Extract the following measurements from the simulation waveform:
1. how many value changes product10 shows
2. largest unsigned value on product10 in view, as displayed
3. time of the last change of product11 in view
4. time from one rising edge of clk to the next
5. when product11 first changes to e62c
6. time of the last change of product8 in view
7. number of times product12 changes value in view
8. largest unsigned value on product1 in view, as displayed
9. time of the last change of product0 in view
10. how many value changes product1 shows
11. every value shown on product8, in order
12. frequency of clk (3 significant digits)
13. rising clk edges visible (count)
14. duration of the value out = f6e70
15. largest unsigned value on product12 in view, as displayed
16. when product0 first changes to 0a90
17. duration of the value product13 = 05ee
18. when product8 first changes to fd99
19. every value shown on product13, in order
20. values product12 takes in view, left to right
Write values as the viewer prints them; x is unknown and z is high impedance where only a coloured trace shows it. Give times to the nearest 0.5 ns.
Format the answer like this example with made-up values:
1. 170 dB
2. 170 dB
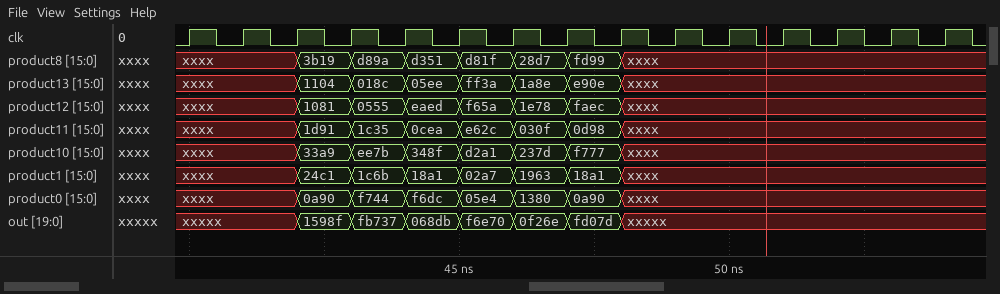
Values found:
1. 7
2. f777
3. 48 ns
4. 1 ns
5. 45 ns
6. 48 ns
7. 7
8. 24c1
9. 48 ns
10. 7
11. xxxx, 3b19, d89a, d351, d81f, 28d7, fd99, xxxx
12. 1.00 GHz
13. 15
14. 1 ns
15. faec
16. 42 ns
17. 1 ns
18. 47 ns
19. xxxx, 1104, 018c, 05ee, ff3a, 1a8e, e90e, xxxx
20. xxxx, 1081, 0555, eaed, f65a, 1e78, faec, xxxx
